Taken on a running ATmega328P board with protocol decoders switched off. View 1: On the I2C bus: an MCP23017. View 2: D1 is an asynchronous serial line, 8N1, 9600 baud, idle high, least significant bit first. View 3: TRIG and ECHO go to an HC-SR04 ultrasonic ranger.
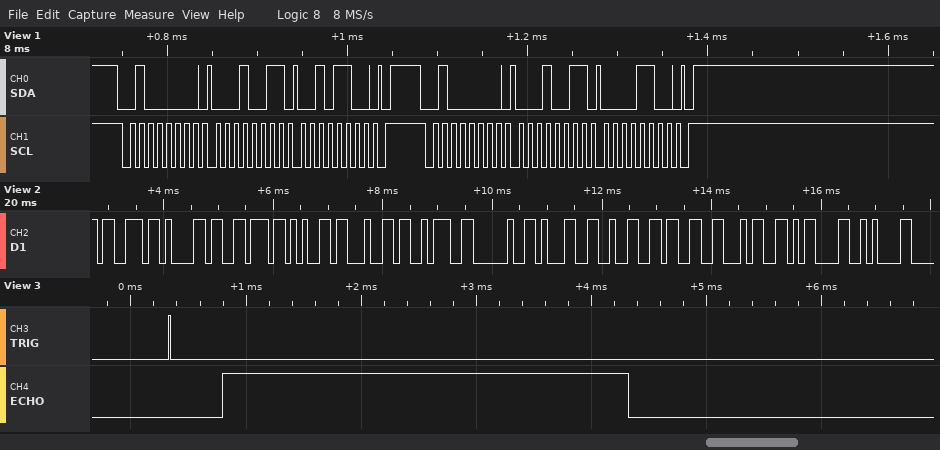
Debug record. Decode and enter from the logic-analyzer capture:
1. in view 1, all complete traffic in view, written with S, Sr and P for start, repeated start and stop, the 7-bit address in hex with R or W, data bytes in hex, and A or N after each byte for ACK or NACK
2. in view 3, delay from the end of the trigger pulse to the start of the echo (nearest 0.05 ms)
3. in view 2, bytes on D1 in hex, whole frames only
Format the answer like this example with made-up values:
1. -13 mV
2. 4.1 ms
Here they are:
1. S 20W A 13 A 2C A P S 20W A 13 A 0C A P
2. 0.45 ms
3. 73 61 76 65 64 3A 20 31 32 33 34 0D 0A
